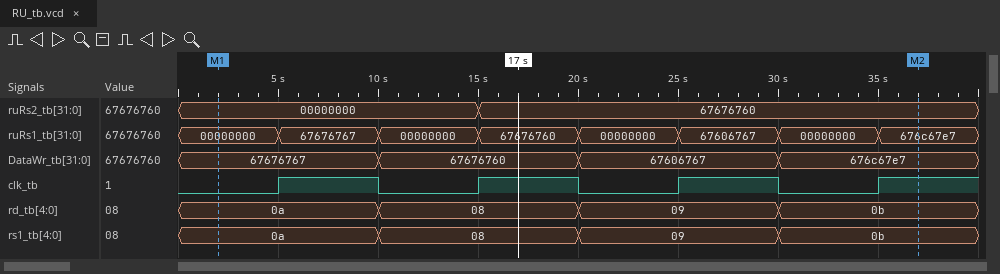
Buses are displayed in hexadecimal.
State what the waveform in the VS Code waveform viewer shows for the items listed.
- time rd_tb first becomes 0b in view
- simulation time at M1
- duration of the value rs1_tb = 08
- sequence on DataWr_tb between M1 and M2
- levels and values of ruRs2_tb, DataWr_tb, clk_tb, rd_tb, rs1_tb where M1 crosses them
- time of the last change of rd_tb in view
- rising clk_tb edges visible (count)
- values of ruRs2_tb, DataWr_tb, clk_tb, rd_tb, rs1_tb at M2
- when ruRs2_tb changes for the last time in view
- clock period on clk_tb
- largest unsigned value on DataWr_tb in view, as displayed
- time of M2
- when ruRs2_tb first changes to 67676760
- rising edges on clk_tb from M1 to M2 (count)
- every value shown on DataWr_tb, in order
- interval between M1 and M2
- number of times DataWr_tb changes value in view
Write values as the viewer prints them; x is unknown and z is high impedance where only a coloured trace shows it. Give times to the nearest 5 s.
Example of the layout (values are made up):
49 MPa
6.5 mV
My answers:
30 s
0 s
10 s
67676767, 67676760, 67606767, 676c67e7
ruRs2_tb=00000000, DataWr_tb=67676767, clk_tb=0, rd_tb=0a, rs1_tb=0a
30 s
4
ruRs2_tb=67676760, DataWr_tb=676c67e7, clk_tb=1, rd_tb=0b, rs1_tb=0b
15 s
10 s
676c67e7
35 s
15 s
4
67676767, 67676760, 67606767, 676c67e7
35 s
3
